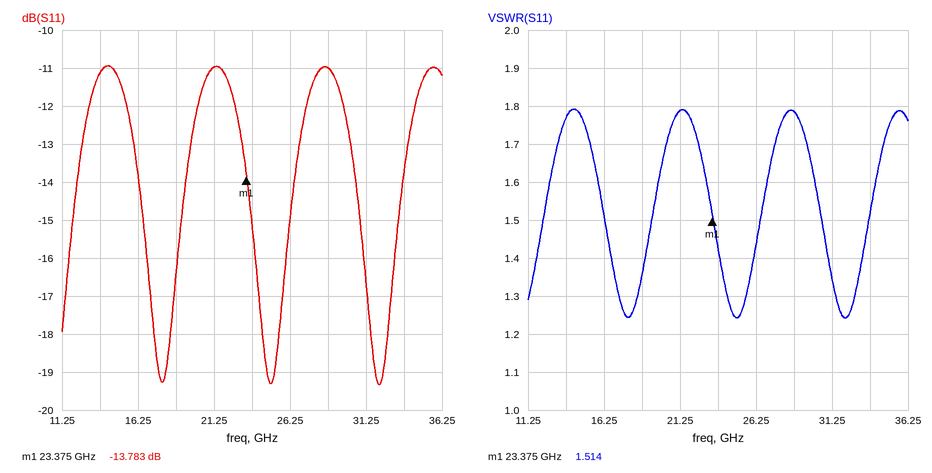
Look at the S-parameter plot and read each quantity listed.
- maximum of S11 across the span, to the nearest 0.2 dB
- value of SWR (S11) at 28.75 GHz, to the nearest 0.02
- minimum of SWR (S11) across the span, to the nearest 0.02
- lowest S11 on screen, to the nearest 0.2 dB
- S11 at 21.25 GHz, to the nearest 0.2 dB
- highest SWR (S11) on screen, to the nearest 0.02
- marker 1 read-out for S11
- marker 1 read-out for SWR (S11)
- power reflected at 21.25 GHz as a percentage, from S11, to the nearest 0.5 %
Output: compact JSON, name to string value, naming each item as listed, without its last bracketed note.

{"maximum of S11 across the span, to the nearest 0.2 dB": "-11.0 dB", "value of SWR (S11) at 28.75 GHz, to the nearest 0.02": "1.78", "minimum of SWR (S11) across the span, to the nearest 0.02": "1.24", "lowest S11 on screen, to the nearest 0.2 dB": "-19.4 dB", "S11 at 21.25 GHz, to the nearest 0.2 dB": "-11.0 dB", "highest SWR (S11) on screen, to the nearest 0.02": "1.80", "marker 1 read-out for S11": "-13.783 dB", "marker 1 read-out for SWR": "1.514", "power reflected at 21.25 GHz as a percentage, from S11, to the nearest 0.5 %": "8.0 %"}
